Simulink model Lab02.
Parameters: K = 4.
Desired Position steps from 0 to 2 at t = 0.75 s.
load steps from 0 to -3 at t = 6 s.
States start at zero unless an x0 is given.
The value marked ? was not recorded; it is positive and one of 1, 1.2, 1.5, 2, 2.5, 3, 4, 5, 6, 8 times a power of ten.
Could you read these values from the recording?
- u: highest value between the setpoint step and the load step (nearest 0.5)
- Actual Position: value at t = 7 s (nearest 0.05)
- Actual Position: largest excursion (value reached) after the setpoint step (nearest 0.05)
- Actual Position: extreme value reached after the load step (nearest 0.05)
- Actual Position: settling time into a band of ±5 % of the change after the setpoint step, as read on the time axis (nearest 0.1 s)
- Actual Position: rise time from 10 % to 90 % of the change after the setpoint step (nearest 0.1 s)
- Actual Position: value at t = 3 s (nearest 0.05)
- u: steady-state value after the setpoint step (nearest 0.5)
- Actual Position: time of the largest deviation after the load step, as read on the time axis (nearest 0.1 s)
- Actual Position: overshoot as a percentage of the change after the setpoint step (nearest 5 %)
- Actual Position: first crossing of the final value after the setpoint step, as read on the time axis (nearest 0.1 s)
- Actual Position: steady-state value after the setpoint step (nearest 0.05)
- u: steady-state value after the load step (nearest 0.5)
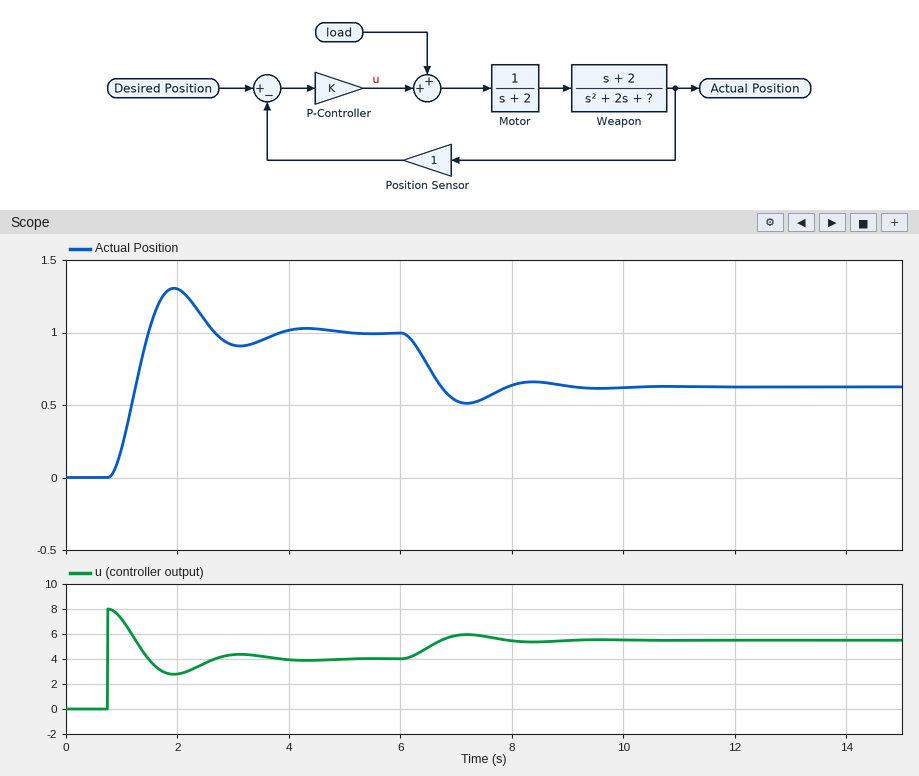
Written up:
8.0
0.55
1.30
0.50
3.5 s
0.5 s
0.90
4.0
7.2 s
30 %
1.5 s
1.00
5.5
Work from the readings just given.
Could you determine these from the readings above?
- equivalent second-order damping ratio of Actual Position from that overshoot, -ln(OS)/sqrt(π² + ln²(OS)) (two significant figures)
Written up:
0.36
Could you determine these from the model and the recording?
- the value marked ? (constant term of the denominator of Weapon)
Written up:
4
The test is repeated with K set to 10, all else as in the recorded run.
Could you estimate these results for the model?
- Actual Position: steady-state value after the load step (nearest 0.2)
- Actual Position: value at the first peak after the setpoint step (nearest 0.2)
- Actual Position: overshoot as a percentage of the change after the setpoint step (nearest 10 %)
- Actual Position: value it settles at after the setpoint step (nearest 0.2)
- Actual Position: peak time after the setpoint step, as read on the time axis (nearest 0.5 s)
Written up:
1.2
2.0
40 %
1.4
1.5 s
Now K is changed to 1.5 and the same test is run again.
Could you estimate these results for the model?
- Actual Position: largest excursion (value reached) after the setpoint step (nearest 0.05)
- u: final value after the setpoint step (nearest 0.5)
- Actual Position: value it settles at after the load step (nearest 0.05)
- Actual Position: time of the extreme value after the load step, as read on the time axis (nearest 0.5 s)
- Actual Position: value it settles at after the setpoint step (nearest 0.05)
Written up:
0.65
2.0
0.00
7.5 s
0.55
